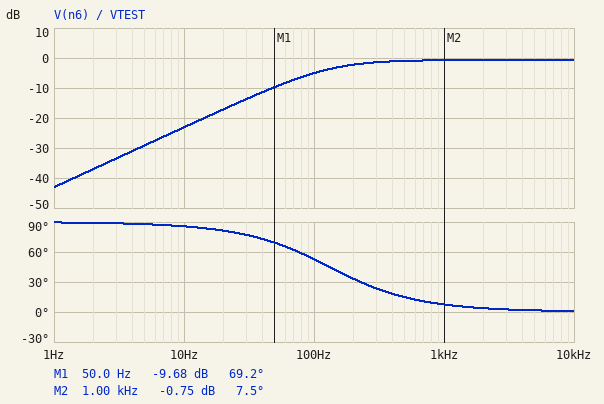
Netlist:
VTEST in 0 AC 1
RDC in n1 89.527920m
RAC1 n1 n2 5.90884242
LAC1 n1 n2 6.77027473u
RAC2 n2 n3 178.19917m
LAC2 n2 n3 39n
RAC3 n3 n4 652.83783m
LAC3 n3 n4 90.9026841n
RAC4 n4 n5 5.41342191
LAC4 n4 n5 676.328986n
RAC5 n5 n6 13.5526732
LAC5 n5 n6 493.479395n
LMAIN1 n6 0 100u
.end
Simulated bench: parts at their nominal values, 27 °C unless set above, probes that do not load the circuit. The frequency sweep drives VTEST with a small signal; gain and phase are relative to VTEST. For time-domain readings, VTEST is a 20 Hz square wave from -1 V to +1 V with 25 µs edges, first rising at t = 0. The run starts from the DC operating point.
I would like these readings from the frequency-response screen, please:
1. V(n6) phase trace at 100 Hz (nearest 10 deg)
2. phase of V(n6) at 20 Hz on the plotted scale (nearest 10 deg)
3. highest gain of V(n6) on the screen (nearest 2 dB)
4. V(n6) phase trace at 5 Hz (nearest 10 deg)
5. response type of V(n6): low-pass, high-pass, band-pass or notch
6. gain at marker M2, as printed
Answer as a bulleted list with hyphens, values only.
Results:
- 50 deg
- 80 deg
- 0 dB
- 90 deg
- high-pass
- -0.75 dB
